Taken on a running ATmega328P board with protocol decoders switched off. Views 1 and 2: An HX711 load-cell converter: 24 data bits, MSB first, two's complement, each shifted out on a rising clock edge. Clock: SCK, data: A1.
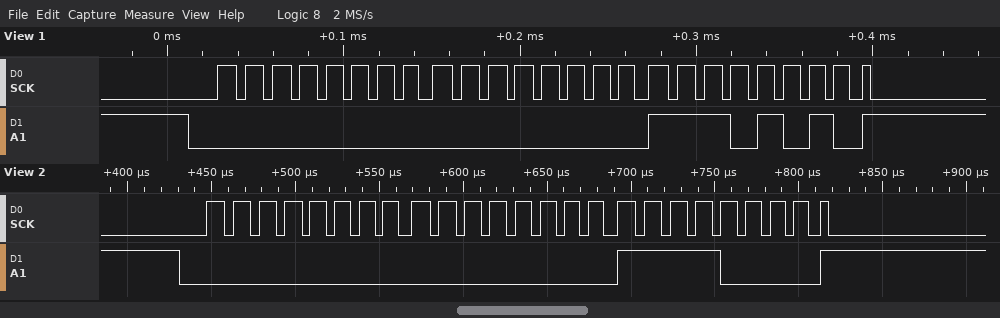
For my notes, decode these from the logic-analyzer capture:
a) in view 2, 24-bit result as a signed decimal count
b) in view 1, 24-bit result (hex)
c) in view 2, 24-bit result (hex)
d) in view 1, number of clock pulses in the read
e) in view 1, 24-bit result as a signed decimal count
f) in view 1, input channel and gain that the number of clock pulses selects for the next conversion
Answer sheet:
240
0x0000EA
0x0000F0
25
234
channel A, gain 128
